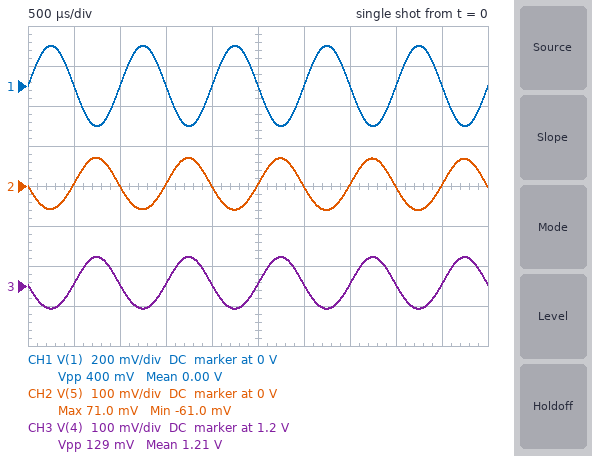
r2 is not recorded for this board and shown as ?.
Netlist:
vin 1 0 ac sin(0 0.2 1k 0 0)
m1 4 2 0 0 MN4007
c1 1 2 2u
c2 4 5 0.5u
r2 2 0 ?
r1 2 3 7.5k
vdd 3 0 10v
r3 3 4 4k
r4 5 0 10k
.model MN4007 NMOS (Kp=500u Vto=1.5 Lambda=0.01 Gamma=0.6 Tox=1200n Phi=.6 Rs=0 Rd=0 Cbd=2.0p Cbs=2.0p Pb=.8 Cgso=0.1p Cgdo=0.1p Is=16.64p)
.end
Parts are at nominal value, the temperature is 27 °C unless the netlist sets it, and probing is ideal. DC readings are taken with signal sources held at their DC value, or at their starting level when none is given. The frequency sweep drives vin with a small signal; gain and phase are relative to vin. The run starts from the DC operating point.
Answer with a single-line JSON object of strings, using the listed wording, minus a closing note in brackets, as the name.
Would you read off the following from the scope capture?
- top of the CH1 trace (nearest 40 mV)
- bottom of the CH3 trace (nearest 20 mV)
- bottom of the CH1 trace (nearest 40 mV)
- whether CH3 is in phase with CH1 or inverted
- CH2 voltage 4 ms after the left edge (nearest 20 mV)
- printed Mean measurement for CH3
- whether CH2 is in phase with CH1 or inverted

{"top of the CH1 trace": "200 mV", "bottom of the CH3 trace": "1.14 V", "bottom of the CH1 trace": "-200 mV", "whether CH3 is in phase with CH1 or inverted": "inverted", "CH2 voltage 4 ms after the left edge": "0 V", "printed Mean measurement for CH3": "1.21 V", "whether CH2 is in phase with CH1 or inverted": "inverted"}
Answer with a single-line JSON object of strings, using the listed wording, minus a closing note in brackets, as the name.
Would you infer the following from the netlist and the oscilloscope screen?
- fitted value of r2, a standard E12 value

{"fitted value of r2, a standard E12 value": "10 kΩ"}
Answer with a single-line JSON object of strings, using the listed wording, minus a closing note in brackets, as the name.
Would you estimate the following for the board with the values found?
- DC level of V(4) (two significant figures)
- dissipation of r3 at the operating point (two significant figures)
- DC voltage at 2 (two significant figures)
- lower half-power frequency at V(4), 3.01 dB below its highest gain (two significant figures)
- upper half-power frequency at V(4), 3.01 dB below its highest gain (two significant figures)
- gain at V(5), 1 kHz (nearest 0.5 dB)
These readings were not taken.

{"DC level of V(4)": "1.2 V", "dissipation of r3 at the operating point": "19 mW", "DC voltage at 2": "5.7 V", "lower half-power frequency at V(4), 3.01 dB below its highest gain": "17 Hz", "upper half-power frequency at V(4), 3.01 dB below its highest gain": "240 MHz", "gain at V(5), 1 kHz": "-10.0 dB"}
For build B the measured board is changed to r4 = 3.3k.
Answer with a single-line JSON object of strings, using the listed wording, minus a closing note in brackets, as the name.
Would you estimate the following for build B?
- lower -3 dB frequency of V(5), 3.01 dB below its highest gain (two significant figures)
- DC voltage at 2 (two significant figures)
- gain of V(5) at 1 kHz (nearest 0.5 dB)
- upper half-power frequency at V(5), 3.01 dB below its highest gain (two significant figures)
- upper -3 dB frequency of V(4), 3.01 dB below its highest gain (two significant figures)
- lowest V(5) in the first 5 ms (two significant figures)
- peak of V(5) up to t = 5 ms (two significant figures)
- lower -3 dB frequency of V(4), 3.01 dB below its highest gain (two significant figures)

{"lower -3 dB frequency of V(5), 3.01 dB below its highest gain": "86 Hz", "DC voltage at 2": "5.7 V", "gain of V(5) at 1 kHz": "-11.0 dB", "upper half-power frequency at V(5), 3.01 dB below its highest gain": "270 MHz", "upper -3 dB frequency of V(4), 3.01 dB below its highest gain": "230 MHz", "lowest V(5) in the first 5 ms": "-56 mV", "peak of V(5) up to t = 5 ms": "65 mV", "lower -3 dB frequency of V(4), 3.01 dB below its highest gain": "16 Hz"}
